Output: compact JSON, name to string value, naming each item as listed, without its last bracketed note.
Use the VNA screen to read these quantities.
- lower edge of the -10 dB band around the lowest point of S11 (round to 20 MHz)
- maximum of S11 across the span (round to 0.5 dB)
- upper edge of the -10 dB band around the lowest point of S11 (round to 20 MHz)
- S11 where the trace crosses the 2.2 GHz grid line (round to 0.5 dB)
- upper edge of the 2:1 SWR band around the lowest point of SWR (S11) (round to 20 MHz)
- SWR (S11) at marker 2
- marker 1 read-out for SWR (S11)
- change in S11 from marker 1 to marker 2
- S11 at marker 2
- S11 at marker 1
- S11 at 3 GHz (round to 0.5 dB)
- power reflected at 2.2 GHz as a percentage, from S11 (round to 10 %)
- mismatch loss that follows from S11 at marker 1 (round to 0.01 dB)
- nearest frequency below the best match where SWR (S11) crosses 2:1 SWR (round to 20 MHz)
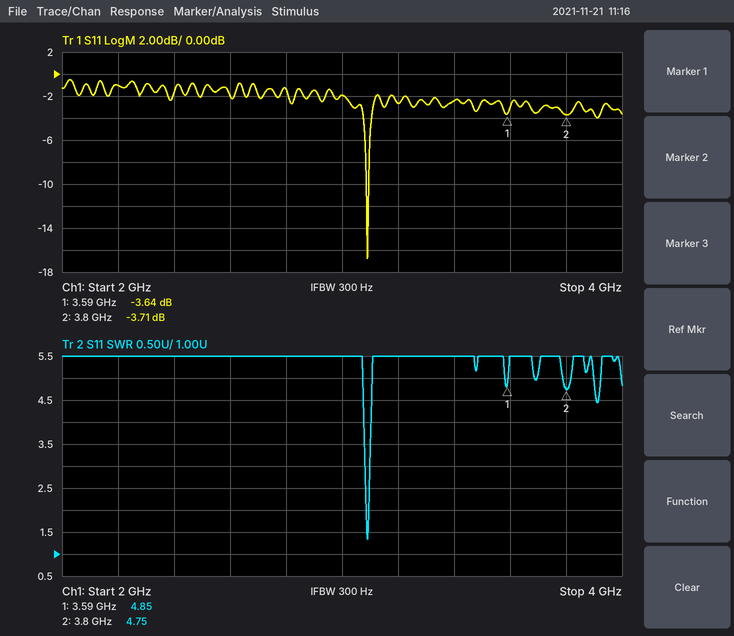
{"lower edge of the -10 dB band around the lowest point of S11": "3.08 GHz", "maximum of S11 across the span": "-0.5 dB", "upper edge of the -10 dB band around the lowest point of S11": "3.10 GHz", "S11 where the trace crosses the 2.2 GHz grid line": "-1.0 dB", "upper edge of the 2:1 SWR band around the lowest point of SWR (S11)": "3.10 GHz", "SWR (S11) at marker 2": "4.75", "marker 1 read-out for SWR": "4.85", "change in S11 from marker 1 to marker 2": "-0.07 dB", "S11 at marker 2": "-3.71 dB", "S11 at marker 1": "-3.64 dB", "S11 at 3 GHz": "-2.0 dB", "power reflected at 2.2 GHz as a percentage, from S11": "80 %", "mismatch loss that follows from S11 at marker 1": "2.46 dB", "nearest frequency below the best match where SWR (S11) crosses 2:1 SWR": "3.08 GHz"}
